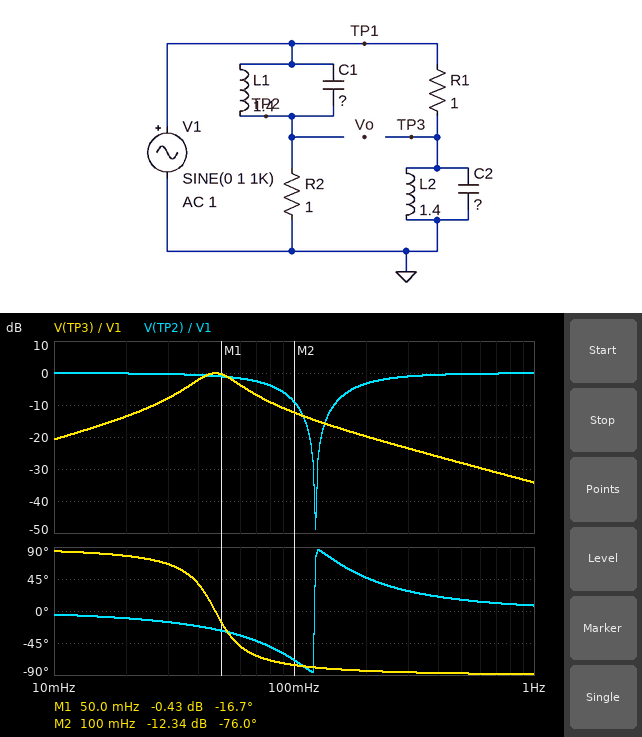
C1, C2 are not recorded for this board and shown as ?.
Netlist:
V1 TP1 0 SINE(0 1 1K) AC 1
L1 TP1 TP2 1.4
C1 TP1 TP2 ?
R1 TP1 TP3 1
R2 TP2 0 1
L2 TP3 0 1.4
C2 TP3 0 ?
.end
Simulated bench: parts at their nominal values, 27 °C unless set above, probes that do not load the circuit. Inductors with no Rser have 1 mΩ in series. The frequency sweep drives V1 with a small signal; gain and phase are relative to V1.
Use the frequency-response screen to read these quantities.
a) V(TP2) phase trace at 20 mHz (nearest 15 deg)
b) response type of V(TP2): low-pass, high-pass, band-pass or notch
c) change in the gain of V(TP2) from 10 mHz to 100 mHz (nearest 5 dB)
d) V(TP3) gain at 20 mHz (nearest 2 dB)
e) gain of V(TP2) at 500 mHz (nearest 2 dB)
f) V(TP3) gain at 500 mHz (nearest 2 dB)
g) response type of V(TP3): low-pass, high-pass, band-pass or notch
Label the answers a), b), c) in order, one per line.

a) -15 deg
b) notch
c) -10 dB
d) -14 dB
e) 0 dB
f) -28 dB
g) band-pass
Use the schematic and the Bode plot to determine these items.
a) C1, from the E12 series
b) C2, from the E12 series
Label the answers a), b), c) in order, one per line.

a) 1.2 F
b) 8.2 F
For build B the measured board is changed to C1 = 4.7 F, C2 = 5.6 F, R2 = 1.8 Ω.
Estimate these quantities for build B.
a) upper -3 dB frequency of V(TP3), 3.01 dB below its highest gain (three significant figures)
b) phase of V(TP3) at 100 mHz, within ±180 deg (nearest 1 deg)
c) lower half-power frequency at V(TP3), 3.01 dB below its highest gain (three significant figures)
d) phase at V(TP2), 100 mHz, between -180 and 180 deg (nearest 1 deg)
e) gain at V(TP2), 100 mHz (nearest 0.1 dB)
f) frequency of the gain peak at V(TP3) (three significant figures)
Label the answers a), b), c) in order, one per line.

a) 72.9 mHz
b) -67 deg
c) 44.4 mHz
d) 17 deg
e) -0.4 dB
f) 56.9 mHz
